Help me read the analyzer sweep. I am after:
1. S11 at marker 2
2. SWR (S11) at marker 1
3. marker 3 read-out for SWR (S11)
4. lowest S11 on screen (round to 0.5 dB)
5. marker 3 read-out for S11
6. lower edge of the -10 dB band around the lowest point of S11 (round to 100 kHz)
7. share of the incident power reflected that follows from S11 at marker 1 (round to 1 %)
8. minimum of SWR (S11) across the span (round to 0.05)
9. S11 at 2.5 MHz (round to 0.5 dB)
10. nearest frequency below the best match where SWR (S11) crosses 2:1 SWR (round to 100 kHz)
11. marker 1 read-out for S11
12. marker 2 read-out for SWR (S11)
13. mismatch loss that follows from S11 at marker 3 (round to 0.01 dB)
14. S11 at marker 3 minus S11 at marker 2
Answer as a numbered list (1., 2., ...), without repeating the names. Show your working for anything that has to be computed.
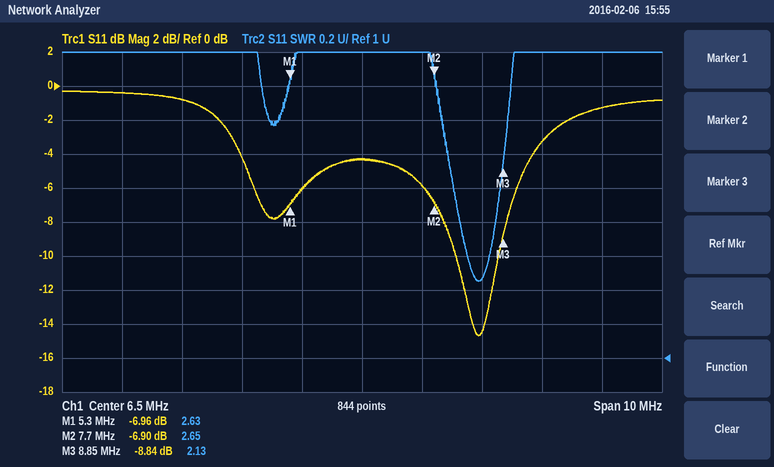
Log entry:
1. -6.90 dB
2. 2.63
3. 2.13
4. -14.5 dB
5. -8.84 dB
6. 8.1 MHz
7. 10^(-6.96/10) ≈ 20 %
8. 1.45
9. -0.5 dB
10. 8.0 MHz
11. -6.96 dB
12. 2.65
13. −10 log10(1 − 10^(-8.84/10)) ≈ 0.61 dB
14. -8.84 − (-6.9) = -1.94 dB
